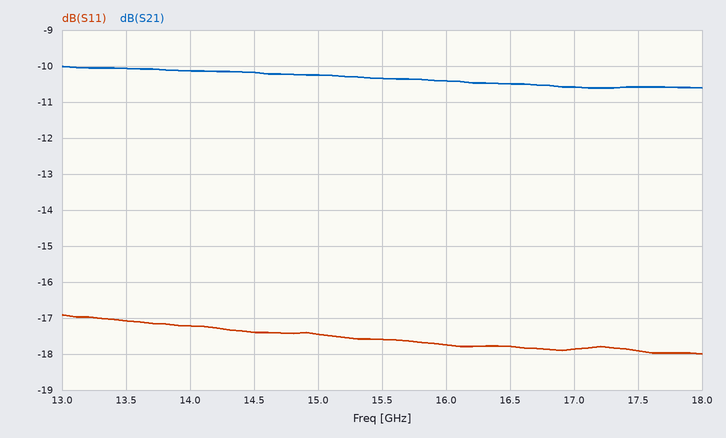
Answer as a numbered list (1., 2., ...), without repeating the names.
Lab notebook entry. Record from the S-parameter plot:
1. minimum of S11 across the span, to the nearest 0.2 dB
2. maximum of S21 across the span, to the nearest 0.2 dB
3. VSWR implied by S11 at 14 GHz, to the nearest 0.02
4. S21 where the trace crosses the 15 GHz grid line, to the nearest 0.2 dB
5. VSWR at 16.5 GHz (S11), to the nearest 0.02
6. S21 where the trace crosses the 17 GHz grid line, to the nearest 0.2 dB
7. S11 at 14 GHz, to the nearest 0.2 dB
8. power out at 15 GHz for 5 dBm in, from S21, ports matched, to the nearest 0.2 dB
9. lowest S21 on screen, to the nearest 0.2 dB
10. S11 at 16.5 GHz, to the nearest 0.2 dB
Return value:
1. -18.0 dB
2. -10.0 dB
3. 1.32
4. -10.2 dB
5. 1.30
6. -10.6 dB
7. -17.2 dB
8. -5.2 dBm
9. -10.6 dB
10. -17.8 dB
